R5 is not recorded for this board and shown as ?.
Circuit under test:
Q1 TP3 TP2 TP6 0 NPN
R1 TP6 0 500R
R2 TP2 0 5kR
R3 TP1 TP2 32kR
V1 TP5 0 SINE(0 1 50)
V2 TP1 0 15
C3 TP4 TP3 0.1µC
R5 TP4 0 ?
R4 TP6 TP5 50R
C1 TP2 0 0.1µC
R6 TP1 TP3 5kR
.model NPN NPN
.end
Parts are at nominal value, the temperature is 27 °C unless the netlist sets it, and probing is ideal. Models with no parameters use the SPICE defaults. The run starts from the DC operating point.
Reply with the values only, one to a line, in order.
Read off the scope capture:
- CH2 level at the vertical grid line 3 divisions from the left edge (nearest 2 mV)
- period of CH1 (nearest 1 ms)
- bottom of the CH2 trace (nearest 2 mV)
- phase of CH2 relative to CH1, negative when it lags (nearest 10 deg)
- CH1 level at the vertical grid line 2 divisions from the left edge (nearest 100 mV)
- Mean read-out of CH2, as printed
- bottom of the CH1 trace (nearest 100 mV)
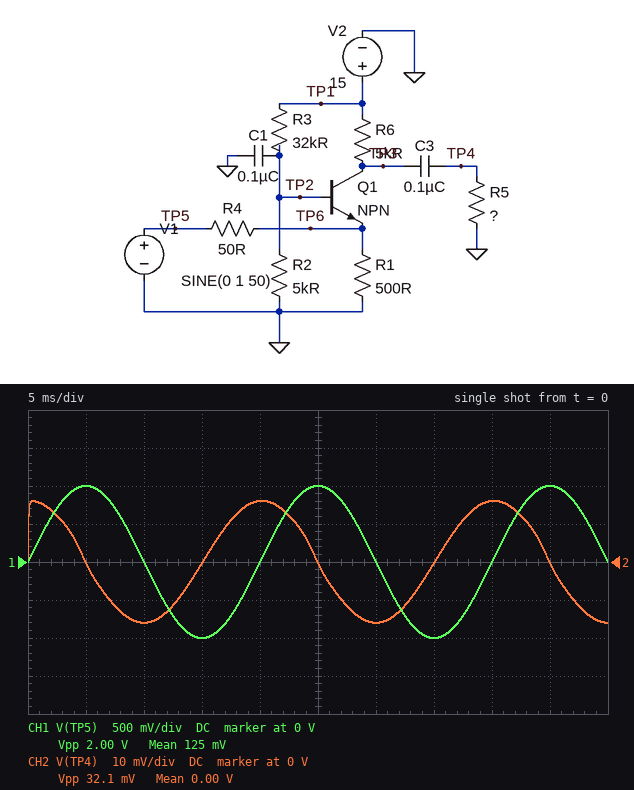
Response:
0 V
20 ms
-16 mV
90 deg
0 V
0.00 V
-1.0 V
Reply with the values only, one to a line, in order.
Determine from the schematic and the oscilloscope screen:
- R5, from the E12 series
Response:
560 Ω
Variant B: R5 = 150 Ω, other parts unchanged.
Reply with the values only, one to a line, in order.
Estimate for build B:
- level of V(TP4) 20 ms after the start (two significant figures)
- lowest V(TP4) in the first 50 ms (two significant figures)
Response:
4.3 mV
-4.3 mV
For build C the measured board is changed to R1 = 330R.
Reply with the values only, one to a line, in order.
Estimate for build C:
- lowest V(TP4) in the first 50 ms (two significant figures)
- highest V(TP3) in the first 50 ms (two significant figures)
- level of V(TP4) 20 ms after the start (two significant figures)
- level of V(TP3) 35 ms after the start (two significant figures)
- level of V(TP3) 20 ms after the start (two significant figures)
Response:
-15 mV
1.1 V
15 mV
-650 mV
210 mV
